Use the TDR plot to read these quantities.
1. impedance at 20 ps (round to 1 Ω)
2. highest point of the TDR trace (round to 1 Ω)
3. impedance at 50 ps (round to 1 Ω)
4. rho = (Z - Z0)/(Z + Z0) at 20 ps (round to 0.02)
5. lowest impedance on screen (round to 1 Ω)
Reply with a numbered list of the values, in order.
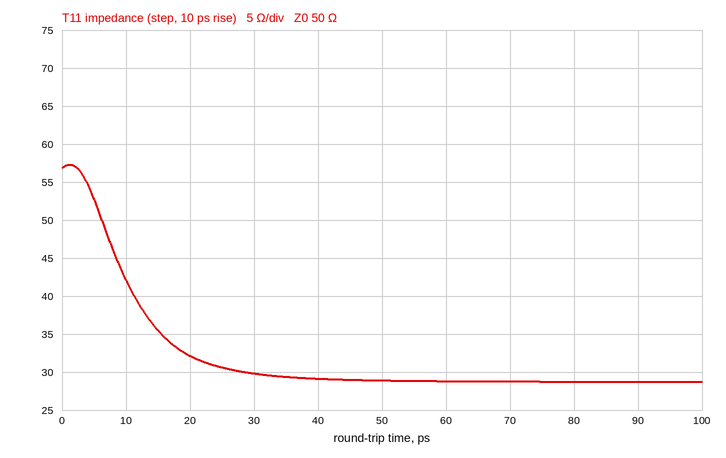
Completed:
1. 32 Ω
2. 57 Ω
3. 29 Ω
4. -0.22
5. 29 Ω
